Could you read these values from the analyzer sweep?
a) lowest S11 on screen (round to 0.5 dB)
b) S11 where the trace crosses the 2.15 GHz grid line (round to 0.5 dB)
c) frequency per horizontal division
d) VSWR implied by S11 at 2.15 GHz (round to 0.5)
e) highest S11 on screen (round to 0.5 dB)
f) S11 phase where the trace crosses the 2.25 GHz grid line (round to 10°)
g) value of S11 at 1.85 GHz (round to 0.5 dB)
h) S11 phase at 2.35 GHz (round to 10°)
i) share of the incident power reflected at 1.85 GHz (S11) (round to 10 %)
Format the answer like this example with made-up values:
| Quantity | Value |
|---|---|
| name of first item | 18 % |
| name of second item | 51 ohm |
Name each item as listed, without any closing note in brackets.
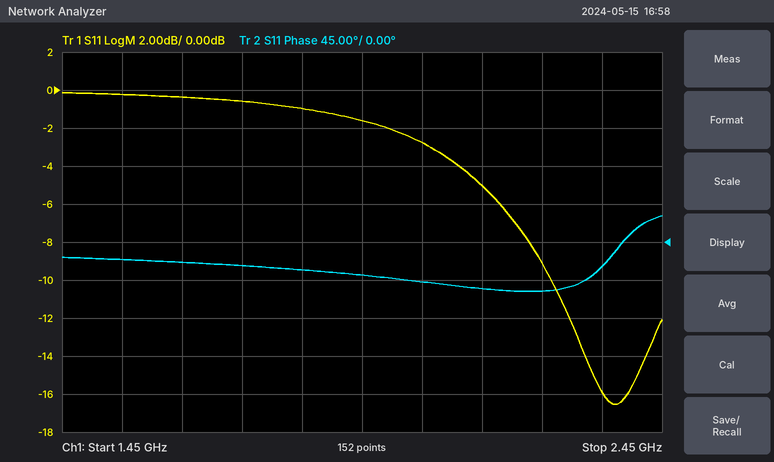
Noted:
| Quantity | Value |
|---|---|
| lowest S11 on screen | -16.5 dB |
| S11 where the trace crosses the 2.15 GHz grid line | -5.0 dB |
| frequency per horizontal division | 100 MHz |
| VSWR implied by S11 at 2.15 GHz | 3.5 |
| highest S11 on screen | 0.0 dB |
| S11 phase where the trace crosses the 2.25 GHz grid line | -60° |
| value of S11 at 1.85 GHz | -1.0 dB |
| S11 phase at 2.35 GHz | -30° |
| share of the incident power reflected at 1.85 GHz (S11) | 80 % |
